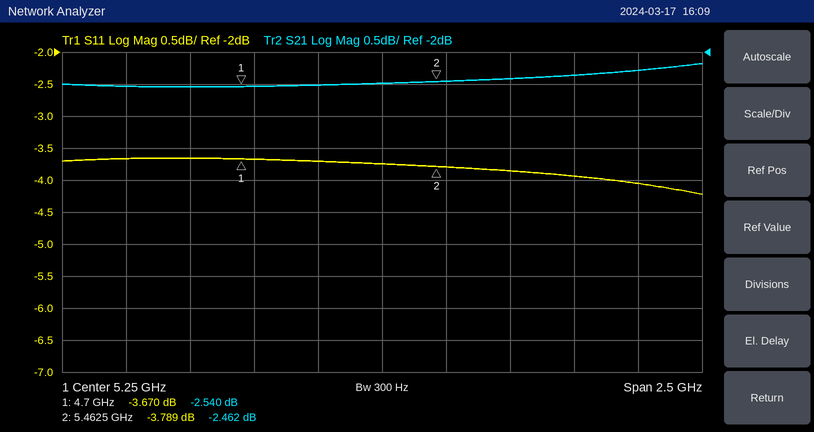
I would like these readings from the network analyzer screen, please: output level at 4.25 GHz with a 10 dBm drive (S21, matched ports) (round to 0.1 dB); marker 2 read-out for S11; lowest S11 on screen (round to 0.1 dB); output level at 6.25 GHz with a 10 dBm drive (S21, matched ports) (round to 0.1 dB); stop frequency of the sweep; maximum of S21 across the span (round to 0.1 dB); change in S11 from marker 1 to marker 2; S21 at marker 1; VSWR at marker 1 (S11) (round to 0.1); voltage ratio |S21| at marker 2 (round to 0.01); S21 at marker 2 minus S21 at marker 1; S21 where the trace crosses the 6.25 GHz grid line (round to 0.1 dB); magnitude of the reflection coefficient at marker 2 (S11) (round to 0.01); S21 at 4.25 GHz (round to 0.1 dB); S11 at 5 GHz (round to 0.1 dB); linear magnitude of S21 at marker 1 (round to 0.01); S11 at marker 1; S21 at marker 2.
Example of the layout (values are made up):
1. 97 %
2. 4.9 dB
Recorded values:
1. 7.5 dBm
2. -3.789 dB
3. -4.2 dB
4. 7.7 dBm
5. 6.5 GHz
6. -2.2 dB
7. -0.119 dB
8. -2.540 dB
9. 4.8
10. 0.75
11. 0.078 dB
12. -2.3 dB
13. 0.65
14. -2.5 dB
15. -3.7 dB
16. 0.75
17. -3.670 dB
18. -2.462 dB
